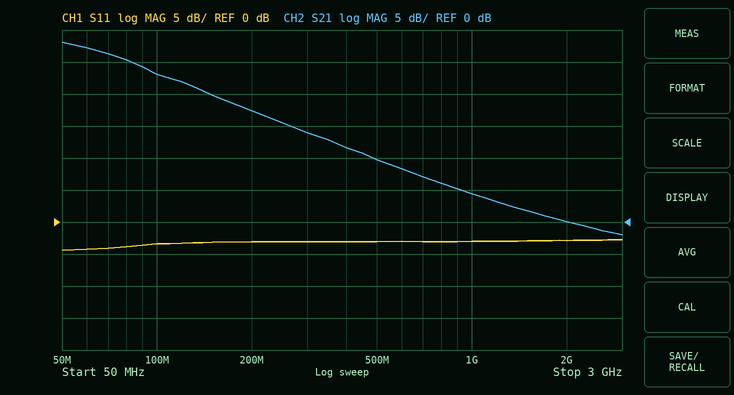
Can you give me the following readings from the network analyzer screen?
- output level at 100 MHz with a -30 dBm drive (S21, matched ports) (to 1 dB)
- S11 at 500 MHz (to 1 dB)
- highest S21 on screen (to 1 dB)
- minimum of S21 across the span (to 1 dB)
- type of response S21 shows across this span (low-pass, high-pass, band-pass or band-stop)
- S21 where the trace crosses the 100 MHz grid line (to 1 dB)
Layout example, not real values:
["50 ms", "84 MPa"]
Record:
["-7 dBm", "-3 dB", "28 dB", "-2 dB", "low-pass", "23 dB"]
